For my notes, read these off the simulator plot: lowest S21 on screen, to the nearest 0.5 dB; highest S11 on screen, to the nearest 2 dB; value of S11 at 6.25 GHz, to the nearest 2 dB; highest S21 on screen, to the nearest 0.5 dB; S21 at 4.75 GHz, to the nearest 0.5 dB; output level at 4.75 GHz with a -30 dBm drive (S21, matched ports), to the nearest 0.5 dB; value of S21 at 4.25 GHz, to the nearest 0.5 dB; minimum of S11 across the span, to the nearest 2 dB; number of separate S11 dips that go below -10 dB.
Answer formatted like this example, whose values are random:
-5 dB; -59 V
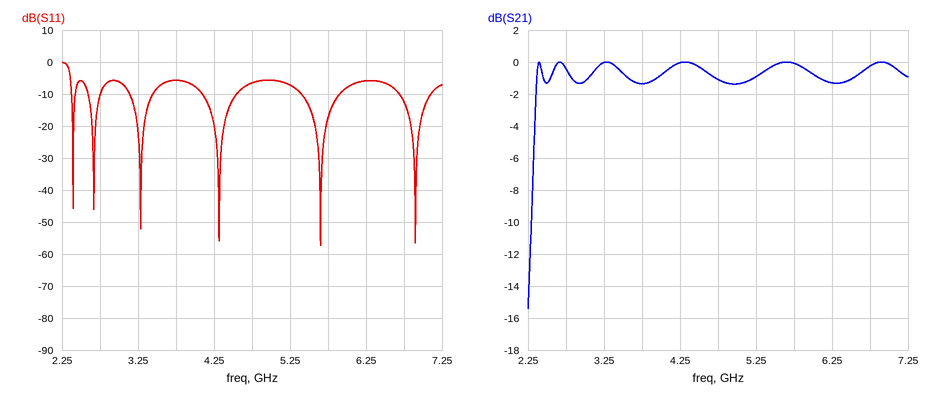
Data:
-15.5 dB; 0 dB; -6 dB; 0.0 dB; -1.0 dB; -31.0 dBm; 0.0 dB; -58 dB; 6
